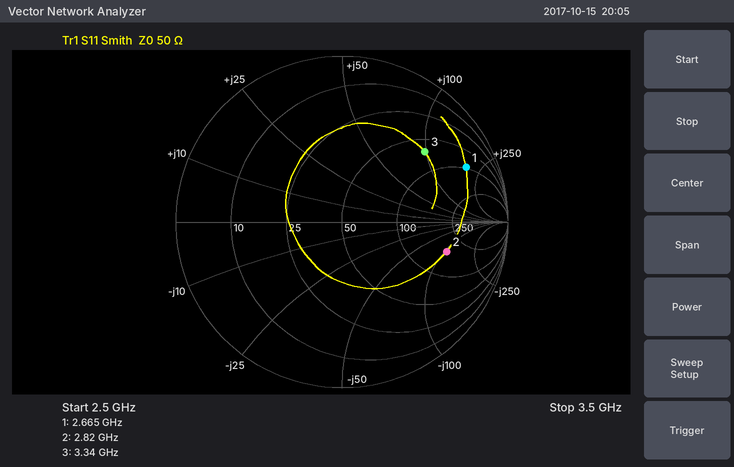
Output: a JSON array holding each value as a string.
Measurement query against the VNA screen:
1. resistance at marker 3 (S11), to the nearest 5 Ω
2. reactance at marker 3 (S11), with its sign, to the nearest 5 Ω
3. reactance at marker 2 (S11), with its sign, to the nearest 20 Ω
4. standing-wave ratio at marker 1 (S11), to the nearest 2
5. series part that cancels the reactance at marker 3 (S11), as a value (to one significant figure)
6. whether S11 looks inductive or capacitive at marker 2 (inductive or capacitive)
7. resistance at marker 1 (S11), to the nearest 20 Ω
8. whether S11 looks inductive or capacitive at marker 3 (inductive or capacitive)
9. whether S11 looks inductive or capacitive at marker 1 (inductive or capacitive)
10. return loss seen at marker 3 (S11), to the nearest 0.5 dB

["65 Ω", "+100 Ω", "-100 Ω", "10", "500 fF", "capacitive", "100 Ω", "inductive", "inductive", "3.5 dB"]
